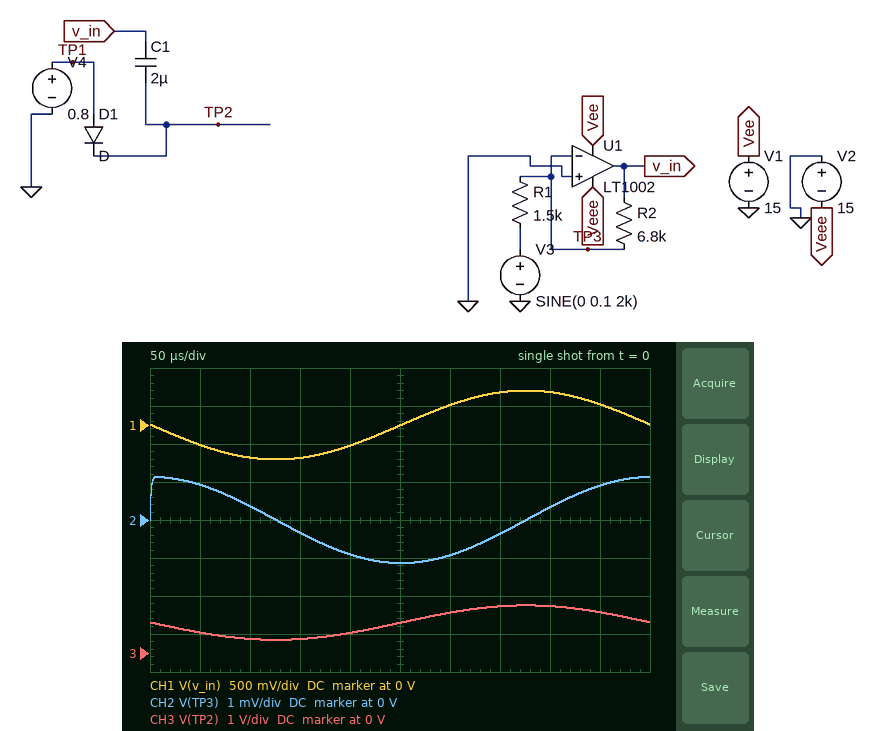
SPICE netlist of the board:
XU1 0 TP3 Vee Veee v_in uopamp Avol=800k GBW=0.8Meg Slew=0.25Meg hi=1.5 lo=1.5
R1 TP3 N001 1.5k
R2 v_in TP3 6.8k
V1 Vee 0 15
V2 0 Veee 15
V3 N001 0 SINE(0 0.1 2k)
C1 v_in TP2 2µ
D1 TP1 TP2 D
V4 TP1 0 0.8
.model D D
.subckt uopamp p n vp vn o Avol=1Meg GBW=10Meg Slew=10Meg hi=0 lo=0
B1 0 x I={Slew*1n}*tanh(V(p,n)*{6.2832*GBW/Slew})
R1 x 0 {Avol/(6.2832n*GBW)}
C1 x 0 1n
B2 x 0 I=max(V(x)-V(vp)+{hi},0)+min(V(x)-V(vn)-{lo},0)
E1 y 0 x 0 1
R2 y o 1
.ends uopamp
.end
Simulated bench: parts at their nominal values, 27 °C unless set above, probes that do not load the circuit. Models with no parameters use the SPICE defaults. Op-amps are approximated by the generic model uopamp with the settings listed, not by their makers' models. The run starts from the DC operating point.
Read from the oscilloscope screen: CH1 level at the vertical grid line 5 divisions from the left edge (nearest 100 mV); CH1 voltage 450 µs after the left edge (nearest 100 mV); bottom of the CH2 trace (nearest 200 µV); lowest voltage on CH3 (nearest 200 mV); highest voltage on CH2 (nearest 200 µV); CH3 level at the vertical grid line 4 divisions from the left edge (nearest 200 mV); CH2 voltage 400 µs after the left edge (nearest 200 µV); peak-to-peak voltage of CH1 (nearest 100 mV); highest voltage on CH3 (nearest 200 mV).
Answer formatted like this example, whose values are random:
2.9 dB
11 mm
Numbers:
0 V
300 mV
-1.2 mV
400 mV
1.2 mV
600 mV
400 µV
900 mV
1.2 V
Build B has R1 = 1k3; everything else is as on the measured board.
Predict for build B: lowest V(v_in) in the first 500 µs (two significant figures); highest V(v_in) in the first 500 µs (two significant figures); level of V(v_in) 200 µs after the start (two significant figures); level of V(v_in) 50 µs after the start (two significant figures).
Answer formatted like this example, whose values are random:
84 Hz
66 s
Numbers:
-520 mV
520 mV
-310 mV
-300 mV
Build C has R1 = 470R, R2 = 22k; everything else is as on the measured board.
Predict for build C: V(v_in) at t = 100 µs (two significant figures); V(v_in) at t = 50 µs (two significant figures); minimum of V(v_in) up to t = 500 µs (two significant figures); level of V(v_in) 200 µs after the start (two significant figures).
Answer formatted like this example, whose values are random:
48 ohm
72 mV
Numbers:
-4.2 V
-2.3 V
-4.7 V
-3.2 V
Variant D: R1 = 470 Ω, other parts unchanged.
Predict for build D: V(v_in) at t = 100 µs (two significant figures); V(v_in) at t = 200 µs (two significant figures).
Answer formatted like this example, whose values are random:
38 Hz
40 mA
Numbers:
-1.4 V
-890 mV
